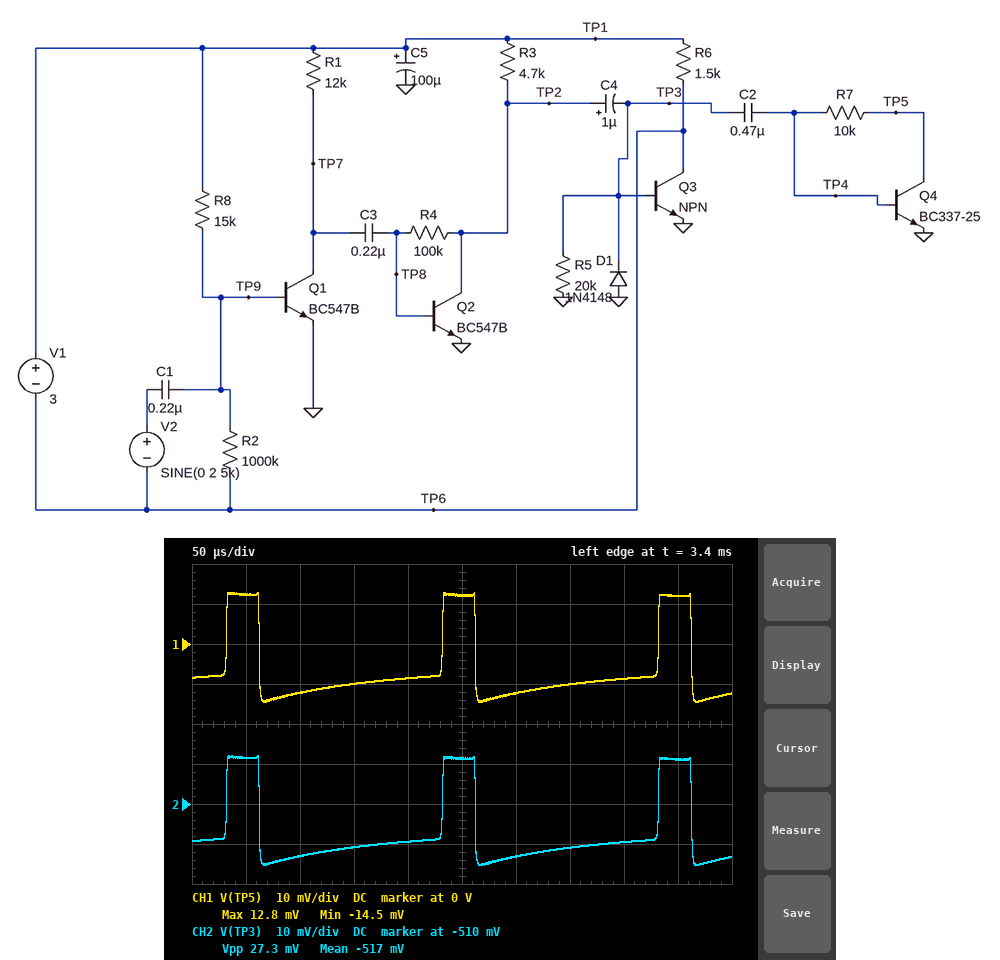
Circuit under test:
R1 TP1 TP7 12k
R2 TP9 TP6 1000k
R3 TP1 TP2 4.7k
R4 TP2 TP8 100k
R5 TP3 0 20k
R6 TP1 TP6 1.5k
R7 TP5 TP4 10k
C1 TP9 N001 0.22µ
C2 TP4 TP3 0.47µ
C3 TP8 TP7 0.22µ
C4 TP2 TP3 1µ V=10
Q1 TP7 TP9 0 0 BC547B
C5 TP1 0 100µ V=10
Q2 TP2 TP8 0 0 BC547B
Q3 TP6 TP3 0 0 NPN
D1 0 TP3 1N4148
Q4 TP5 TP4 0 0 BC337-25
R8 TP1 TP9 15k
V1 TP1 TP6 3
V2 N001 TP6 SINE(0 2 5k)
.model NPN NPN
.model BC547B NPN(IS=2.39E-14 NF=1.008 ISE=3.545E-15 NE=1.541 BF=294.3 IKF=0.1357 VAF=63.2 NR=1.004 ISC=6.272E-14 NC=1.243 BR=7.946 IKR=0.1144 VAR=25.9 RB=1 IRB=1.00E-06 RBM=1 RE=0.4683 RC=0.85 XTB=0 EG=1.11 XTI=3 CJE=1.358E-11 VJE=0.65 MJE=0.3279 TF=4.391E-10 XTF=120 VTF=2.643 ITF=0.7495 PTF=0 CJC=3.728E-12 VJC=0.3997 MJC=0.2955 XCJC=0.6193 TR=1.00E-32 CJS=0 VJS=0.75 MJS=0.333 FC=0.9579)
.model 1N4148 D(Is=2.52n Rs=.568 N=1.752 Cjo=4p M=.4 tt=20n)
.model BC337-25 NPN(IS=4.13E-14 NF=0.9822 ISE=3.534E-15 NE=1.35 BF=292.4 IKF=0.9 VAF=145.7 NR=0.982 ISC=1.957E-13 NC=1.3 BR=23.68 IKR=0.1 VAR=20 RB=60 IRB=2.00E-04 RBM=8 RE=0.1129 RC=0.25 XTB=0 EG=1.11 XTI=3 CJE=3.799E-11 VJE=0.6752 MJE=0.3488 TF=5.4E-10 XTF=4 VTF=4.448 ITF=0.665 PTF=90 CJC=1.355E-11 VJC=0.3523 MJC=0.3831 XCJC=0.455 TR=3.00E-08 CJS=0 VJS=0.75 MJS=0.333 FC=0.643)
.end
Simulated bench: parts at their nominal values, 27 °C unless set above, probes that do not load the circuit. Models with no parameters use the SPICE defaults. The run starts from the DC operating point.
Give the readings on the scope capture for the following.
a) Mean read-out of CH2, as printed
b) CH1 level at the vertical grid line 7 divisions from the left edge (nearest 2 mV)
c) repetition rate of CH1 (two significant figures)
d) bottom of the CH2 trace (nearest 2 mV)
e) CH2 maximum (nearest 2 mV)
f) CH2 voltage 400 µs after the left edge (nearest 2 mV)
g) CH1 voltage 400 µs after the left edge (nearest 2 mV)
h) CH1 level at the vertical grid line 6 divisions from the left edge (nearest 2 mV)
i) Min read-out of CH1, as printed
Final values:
-517 mV
-10 mV
5.0 kHz
-526 mV
-498 mV
-520 mV
-8 mV
-12 mV
-14.5 mV
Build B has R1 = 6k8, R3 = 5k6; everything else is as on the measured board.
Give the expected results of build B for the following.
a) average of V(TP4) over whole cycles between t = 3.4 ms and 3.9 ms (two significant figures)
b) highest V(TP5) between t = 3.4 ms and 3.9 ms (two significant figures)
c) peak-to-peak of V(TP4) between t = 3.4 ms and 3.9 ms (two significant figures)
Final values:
-4.2 mV
11 mV
21 mV
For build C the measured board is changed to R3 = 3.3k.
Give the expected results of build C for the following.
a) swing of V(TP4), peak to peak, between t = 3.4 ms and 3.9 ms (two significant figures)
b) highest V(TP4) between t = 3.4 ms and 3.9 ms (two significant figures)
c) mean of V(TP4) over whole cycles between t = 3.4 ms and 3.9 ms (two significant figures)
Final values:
32 mV
14 mV
-8.2 mV
